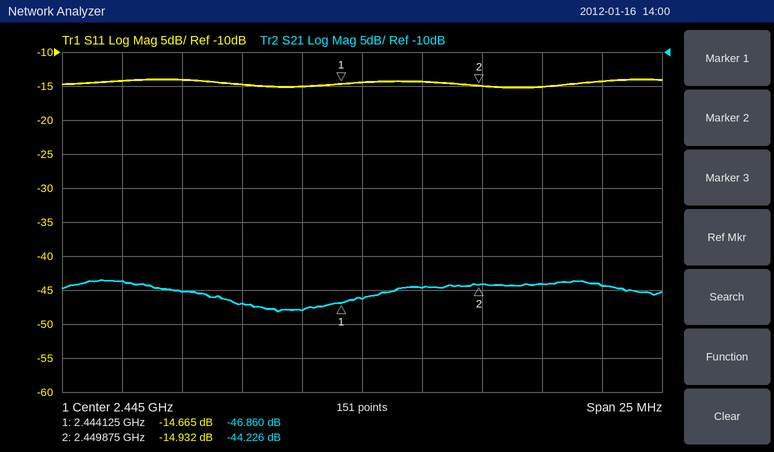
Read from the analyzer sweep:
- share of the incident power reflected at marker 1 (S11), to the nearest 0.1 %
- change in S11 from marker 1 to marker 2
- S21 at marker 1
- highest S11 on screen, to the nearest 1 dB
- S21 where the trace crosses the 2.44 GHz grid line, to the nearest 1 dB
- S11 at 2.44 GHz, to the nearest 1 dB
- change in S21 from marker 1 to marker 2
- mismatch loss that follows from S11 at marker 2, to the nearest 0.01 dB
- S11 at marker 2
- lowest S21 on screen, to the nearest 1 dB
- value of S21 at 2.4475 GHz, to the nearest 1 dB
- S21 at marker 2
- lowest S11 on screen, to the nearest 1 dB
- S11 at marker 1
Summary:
3.4 %
-0.267 dB
-46.860 dB
-14 dB
-47 dB
-15 dB
2.634 dB
0.14 dB
-14.932 dB
-48 dB
-45 dB
-44.226 dB
-15 dB
-14.665 dB
